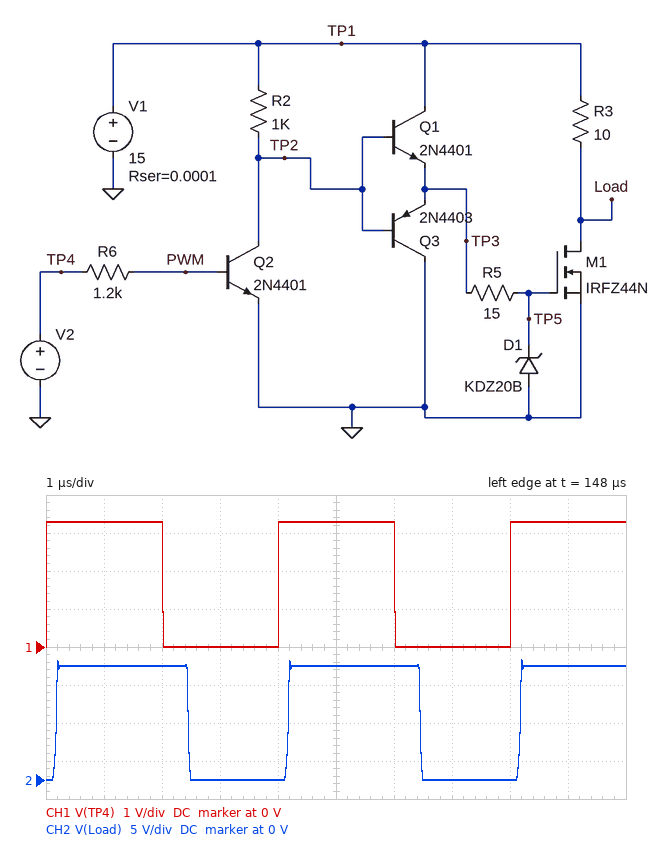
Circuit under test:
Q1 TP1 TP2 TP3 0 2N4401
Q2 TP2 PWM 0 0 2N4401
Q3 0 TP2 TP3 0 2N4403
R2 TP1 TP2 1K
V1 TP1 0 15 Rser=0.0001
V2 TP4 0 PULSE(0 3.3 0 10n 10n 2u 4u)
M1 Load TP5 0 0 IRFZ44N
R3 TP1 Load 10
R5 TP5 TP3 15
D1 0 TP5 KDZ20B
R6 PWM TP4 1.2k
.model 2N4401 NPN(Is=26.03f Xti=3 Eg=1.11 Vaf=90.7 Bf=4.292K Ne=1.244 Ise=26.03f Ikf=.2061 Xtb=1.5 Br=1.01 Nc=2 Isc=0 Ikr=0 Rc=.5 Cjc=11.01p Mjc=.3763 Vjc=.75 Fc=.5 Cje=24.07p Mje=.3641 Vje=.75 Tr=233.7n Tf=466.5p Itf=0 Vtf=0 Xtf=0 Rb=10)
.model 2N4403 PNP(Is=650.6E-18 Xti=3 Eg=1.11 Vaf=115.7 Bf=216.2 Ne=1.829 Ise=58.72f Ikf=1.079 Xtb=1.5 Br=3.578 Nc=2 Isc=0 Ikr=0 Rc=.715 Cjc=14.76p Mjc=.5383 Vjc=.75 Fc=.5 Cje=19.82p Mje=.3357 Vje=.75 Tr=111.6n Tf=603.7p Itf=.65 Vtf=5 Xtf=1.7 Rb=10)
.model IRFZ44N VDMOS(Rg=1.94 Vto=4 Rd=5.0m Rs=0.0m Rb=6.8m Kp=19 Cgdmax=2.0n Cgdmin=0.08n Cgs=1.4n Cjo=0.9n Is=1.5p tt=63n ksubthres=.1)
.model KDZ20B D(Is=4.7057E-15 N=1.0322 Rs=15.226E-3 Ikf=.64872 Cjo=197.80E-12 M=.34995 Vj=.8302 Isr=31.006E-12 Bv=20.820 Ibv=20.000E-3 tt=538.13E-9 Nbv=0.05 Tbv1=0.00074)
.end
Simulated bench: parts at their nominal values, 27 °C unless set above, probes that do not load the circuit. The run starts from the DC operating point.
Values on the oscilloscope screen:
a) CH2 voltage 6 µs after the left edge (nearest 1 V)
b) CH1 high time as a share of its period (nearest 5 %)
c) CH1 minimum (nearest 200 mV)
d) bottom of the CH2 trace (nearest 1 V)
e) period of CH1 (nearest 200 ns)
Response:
15 V
50 %
0 V
0 V
4.0 µs
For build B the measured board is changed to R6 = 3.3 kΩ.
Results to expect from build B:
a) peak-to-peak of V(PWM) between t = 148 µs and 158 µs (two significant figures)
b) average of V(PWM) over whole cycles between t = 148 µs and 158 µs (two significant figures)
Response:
710 mV
490 mV
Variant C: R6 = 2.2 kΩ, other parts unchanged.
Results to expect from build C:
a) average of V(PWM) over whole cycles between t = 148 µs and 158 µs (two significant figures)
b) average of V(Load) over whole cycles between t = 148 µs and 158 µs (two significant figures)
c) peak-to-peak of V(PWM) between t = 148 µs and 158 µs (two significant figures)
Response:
470 mV
8.6 V
720 mV
